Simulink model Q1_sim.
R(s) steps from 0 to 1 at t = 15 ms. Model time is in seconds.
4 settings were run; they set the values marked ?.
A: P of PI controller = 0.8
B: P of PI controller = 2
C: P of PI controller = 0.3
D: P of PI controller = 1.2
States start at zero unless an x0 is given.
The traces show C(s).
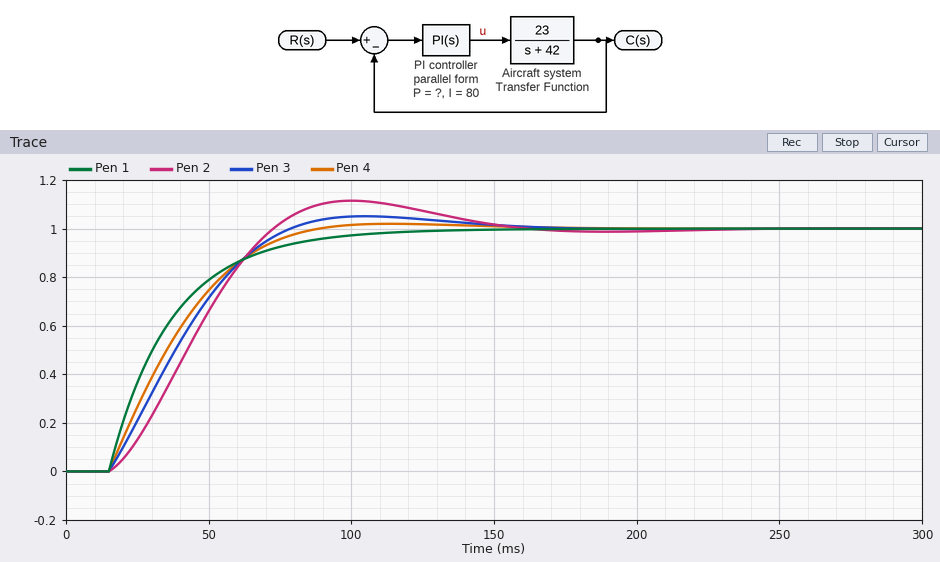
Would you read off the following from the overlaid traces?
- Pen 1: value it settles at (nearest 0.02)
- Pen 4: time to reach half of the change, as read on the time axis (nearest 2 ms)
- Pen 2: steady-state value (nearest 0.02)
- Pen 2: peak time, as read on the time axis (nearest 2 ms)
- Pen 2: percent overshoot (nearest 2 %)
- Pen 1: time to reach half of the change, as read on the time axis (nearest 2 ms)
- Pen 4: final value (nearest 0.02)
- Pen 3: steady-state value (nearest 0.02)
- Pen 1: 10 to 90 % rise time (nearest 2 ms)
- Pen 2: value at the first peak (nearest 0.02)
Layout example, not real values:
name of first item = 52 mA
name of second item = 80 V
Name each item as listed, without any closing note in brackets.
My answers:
Pen 1: value it settles at = 1.00
Pen 4: time to reach half of the change, as read on the time axis = 36 ms
Pen 2: steady-state value = 1.00
Pen 2: peak time, as read on the time axis = 100 ms
Pen 2: percent overshoot = 12 %
Pen 1: time to reach half of the change, as read on the time axis = 30 ms
Pen 4: final value = 1.00
Pen 3: steady-state value = 1.00
Pen 1: 10 to 90 % rise time = 50 ms
Pen 2: value at the first peak = 1.12
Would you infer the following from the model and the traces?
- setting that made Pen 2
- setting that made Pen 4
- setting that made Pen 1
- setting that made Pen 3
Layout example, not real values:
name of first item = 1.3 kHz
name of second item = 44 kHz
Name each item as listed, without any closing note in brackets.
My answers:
setting that made Pen 2 = C
setting that made Pen 4 = D
setting that made Pen 1 = B
setting that made Pen 3 = A
